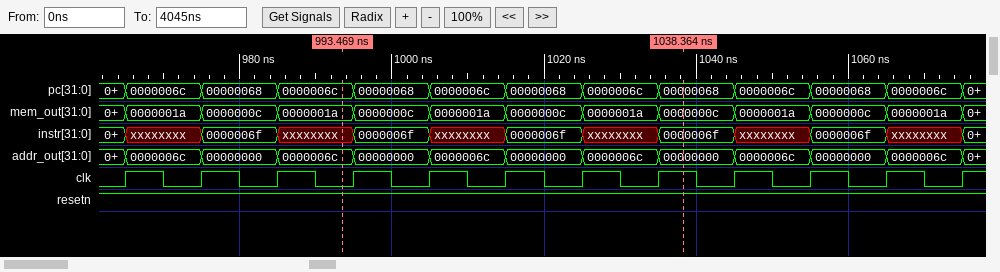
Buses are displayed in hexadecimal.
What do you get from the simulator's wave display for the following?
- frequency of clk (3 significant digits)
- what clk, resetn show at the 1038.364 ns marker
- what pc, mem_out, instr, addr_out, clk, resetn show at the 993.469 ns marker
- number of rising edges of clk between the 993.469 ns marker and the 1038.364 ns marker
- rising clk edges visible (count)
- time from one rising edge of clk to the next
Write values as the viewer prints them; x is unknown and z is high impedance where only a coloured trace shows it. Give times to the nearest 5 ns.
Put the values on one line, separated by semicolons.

100 MHz; clk=1, resetn=1; pc=0000006c, mem_out=0000001a, instr=xxxxxxxx, addr_out=0000006c, clk=0, resetn=1; 5; 12; 10 ns
